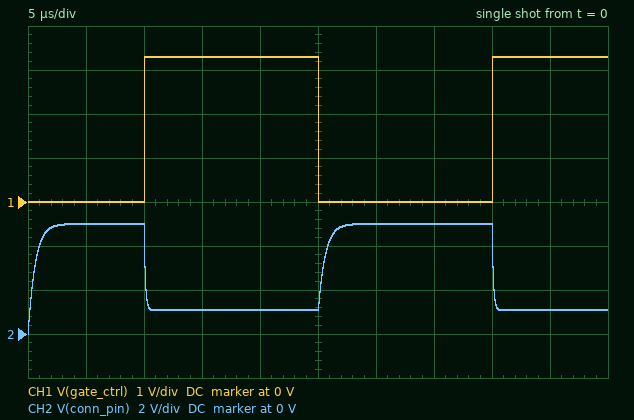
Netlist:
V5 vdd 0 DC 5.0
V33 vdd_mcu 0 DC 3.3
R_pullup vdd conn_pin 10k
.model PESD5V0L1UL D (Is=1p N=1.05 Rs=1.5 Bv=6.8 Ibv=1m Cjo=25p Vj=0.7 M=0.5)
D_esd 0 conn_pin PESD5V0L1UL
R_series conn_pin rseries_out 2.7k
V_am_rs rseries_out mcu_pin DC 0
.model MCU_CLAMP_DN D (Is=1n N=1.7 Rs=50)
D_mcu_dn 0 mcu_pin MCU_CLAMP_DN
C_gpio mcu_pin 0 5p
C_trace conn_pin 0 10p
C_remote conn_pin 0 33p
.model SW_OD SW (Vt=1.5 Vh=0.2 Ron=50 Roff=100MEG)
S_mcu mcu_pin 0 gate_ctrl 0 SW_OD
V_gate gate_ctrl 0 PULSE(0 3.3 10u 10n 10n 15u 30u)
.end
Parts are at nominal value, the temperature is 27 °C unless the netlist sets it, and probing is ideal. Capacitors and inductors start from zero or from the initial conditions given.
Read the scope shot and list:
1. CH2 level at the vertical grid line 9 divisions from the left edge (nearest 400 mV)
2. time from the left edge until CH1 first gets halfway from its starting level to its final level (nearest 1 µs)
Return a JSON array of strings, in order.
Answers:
["1.2 V", "10 µs"]
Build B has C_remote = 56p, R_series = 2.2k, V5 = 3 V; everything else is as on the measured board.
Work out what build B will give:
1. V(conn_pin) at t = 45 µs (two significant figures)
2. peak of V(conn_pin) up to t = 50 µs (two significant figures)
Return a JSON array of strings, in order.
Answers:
["550 mV", "3.0 V"]
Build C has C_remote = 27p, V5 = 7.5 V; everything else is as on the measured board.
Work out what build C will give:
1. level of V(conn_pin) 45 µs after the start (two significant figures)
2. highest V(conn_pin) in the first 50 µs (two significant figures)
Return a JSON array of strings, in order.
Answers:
["1.6 V", "6.7 V"]
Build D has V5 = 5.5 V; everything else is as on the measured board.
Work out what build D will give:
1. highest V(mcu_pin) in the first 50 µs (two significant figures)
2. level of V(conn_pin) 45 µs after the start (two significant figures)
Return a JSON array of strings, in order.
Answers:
["5.5 V", "1.2 V"]
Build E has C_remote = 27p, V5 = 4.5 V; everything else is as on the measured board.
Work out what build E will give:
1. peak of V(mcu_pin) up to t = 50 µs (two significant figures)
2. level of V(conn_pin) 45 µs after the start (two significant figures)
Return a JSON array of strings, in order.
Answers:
["4.5 V", "970 mV"]
